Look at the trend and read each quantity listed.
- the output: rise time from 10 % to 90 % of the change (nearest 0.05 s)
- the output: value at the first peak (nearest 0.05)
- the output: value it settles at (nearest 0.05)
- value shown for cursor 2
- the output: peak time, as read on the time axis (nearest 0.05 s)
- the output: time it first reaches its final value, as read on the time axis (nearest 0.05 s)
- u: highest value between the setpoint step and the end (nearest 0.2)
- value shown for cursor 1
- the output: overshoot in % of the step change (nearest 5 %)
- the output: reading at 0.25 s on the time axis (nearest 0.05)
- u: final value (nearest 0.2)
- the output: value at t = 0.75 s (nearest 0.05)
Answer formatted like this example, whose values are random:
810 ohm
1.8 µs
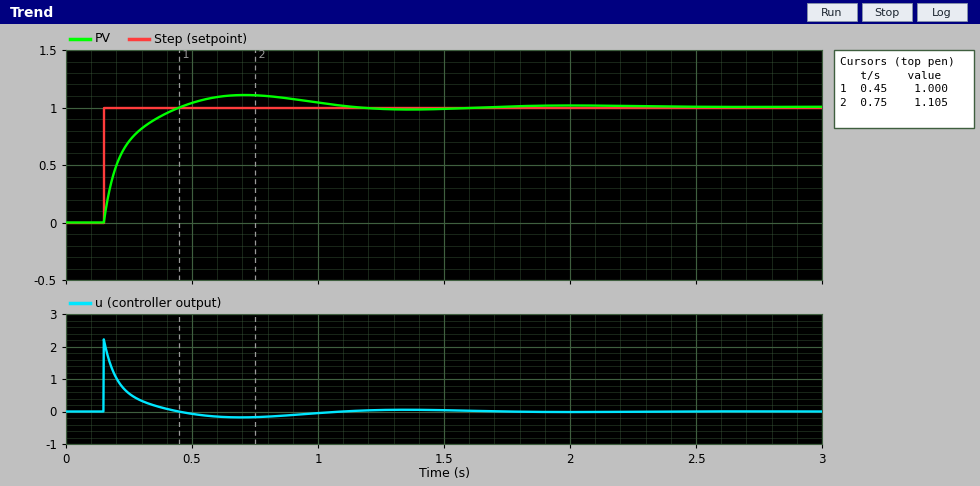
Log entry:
0.20 s
1.10
1.00
1.105
0.70 s
0.45 s
2.2
1.000
10 %
0.70
0.0
1.10
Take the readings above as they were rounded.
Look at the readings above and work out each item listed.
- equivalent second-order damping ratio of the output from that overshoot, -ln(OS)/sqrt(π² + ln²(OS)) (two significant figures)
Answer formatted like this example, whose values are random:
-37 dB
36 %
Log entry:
0.59
